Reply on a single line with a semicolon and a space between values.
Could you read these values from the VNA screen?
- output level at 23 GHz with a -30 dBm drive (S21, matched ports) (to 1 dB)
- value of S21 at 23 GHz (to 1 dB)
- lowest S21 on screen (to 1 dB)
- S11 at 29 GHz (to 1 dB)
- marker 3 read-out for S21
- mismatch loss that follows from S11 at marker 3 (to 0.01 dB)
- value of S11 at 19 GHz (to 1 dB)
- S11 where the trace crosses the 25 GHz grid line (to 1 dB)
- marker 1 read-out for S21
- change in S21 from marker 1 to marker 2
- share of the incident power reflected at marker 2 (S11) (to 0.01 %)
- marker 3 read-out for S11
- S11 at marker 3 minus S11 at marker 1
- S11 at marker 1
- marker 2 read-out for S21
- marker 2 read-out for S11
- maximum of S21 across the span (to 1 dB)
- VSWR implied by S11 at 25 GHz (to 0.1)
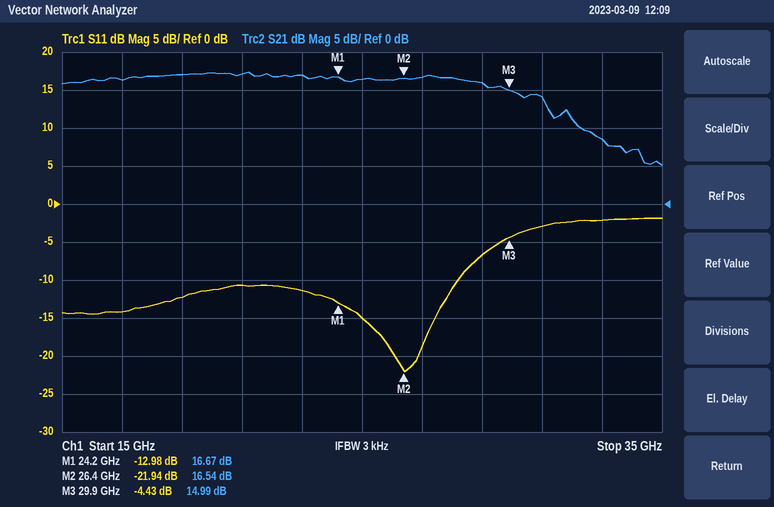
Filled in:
-13 dBm; 17 dB; 5 dB; -7 dB; 14.99 dB; 1.94 dB; -12 dB; -15 dB; 16.67 dB; -0.13 dB; 0.64 %; -4.43 dB; 8.55 dB; -12.98 dB; 16.54 dB; -21.94 dB; 17 dB; 1.4
